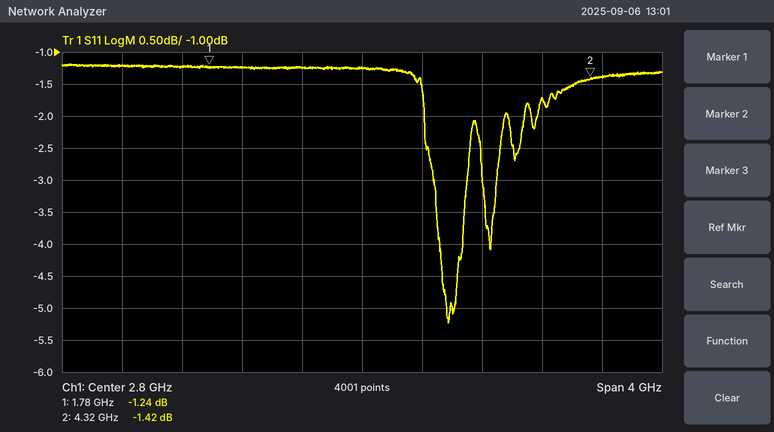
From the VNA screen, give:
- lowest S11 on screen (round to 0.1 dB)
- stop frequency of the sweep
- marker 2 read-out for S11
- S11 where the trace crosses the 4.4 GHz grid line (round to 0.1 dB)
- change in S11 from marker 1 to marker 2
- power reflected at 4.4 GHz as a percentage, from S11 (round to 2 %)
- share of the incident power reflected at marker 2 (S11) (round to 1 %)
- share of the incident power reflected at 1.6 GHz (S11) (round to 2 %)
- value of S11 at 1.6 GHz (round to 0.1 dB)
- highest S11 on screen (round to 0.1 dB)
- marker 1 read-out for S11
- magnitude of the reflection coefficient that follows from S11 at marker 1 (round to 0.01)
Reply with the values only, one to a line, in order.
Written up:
-5.2 dB
4.8 GHz
-1.42 dB
-1.4 dB
-0.18 dB
72 %
72 %
76 %
-1.2 dB
-1.2 dB
-1.24 dB
0.87
